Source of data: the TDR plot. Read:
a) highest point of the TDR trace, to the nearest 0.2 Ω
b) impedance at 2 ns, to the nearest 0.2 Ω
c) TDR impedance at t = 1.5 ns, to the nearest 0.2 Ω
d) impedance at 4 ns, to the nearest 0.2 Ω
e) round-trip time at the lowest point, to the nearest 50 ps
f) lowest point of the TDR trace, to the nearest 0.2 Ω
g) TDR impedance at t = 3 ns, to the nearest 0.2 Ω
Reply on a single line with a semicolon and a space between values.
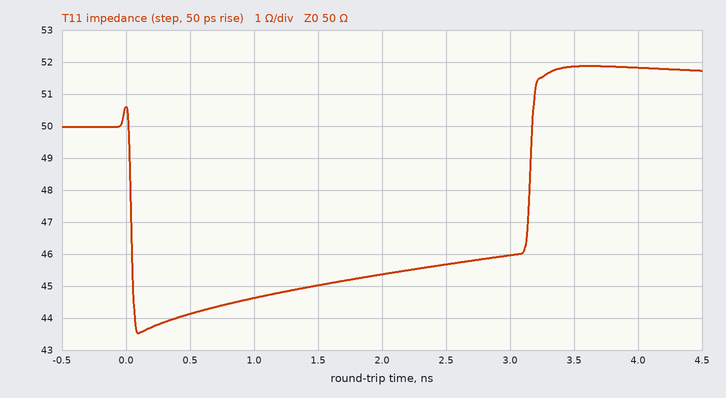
51.8 Ω; 45.4 Ω; 45.0 Ω; 51.8 Ω; 100 ps; 43.6 Ω; 46.0 Ω
